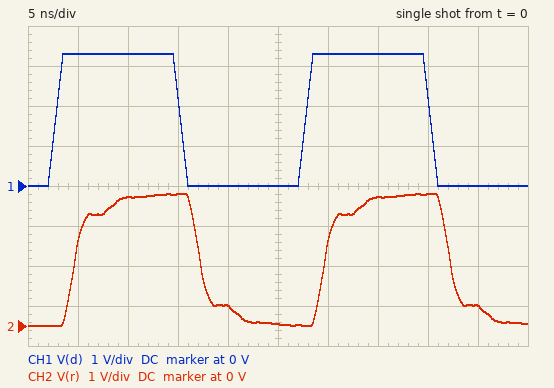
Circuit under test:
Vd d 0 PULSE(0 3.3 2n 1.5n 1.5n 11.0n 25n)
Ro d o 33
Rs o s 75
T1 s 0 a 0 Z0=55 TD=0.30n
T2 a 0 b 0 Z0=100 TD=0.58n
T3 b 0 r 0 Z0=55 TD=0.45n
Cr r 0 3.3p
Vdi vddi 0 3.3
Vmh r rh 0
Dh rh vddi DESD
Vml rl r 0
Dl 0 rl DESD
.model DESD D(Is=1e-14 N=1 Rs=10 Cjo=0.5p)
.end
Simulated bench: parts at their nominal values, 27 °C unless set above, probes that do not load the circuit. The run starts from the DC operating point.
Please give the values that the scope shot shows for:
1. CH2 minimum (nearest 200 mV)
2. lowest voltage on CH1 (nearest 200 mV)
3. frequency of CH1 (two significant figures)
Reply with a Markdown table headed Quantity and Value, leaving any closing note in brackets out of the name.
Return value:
| Quantity | Value |
|---|---|
| CH2 minimum | 0 V |
| lowest voltage on CH1 | 0 V |
| frequency of CH1 | 40 MHz |
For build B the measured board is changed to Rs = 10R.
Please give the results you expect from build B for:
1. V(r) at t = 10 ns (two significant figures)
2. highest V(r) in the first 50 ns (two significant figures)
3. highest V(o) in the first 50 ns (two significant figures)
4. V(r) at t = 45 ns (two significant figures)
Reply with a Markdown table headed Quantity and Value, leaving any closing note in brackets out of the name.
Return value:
| Quantity | Value |
|---|---|
| V(r) at t = 10 ns | 3.1 V |
| highest V(r) in the first 50 ns | 4.1 V |
| highest V(o) in the first 50 ns | 3.5 V |
| V(r) at t = 45 ns | -400 mV |
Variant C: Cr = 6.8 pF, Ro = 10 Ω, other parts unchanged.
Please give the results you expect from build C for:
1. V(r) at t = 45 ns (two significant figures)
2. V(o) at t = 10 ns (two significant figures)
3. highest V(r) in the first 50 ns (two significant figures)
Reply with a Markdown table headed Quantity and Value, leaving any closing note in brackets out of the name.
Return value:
| Quantity | Value |
|---|---|
| V(r) at t = 45 ns | 200 mV |
| V(o) at t = 10 ns | 3.3 V |
| highest V(r) in the first 50 ns | 3.3 V |
